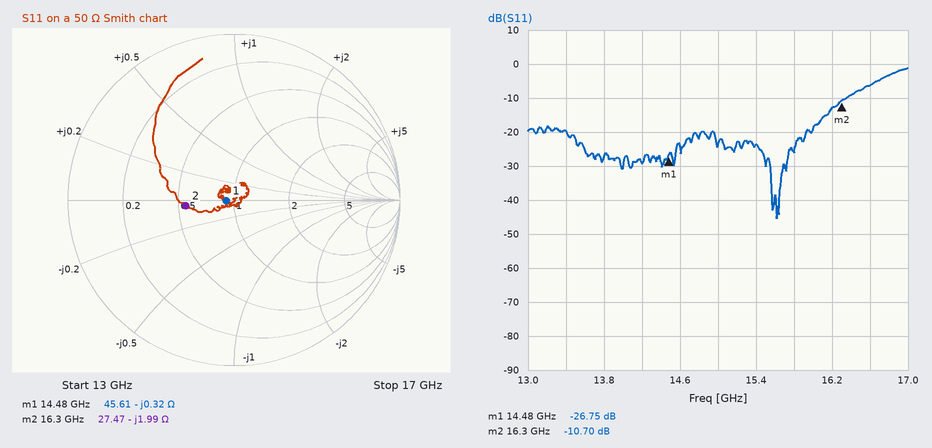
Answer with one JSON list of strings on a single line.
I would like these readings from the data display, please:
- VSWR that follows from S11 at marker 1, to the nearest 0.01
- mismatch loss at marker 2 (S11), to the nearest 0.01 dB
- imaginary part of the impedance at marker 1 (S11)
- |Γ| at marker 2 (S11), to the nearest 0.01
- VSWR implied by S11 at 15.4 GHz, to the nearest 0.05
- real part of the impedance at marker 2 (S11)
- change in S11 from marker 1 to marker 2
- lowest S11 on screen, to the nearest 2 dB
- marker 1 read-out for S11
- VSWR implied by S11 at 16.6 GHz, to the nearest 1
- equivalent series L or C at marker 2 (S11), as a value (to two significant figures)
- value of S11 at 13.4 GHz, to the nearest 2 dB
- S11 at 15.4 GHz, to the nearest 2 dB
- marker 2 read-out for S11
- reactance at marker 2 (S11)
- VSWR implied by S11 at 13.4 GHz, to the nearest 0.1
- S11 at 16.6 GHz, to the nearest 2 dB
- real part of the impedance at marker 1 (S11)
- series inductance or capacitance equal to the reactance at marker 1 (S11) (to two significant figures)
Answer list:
["1.10", "0.39 dB", "-0.32 Ω", "0.29", "1.15", "27.47 Ω", "16.05 dB", "-46 dB", "-26.75 dB", "3", "4.9 pF", "-20 dB", "-24 dB", "-10.70 dB", "-1.99 Ω", "1.2", "-6 dB", "45.61 Ω", "34 pF"]
